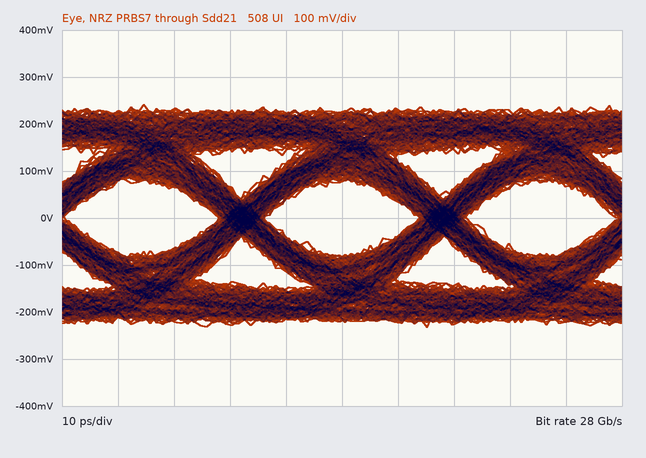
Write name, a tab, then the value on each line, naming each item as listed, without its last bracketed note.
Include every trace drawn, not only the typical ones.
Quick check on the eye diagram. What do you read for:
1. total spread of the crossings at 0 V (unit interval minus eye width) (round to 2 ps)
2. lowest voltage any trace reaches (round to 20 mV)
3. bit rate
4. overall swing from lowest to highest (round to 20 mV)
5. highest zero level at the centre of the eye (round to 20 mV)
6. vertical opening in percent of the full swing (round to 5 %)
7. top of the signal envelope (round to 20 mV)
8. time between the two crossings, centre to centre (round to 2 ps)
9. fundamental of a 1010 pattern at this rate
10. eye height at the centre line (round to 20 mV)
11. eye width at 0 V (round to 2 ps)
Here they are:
total spread of the crossings at 0 V (unit interval minus eye width)	8 ps
lowest voltage any trace reaches	-240 mV
bit rate	28 Gb/s
overall swing from lowest to highest	480 mV
highest zero level at the centre of the eye	-80 mV
vertical opening in percent of the full swing	35 %
top of the signal envelope	240 mV
time between the two crossings, centre to centre	36 ps
fundamental of a 1010 pattern at this rate	14 GHz
eye height at the centre line	160 mV
eye width at 0 V	28 ps
